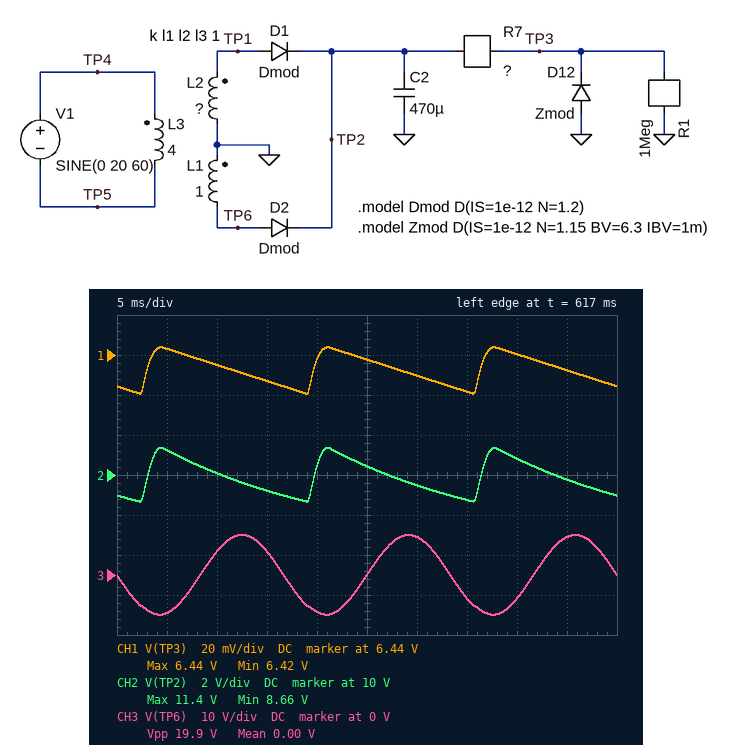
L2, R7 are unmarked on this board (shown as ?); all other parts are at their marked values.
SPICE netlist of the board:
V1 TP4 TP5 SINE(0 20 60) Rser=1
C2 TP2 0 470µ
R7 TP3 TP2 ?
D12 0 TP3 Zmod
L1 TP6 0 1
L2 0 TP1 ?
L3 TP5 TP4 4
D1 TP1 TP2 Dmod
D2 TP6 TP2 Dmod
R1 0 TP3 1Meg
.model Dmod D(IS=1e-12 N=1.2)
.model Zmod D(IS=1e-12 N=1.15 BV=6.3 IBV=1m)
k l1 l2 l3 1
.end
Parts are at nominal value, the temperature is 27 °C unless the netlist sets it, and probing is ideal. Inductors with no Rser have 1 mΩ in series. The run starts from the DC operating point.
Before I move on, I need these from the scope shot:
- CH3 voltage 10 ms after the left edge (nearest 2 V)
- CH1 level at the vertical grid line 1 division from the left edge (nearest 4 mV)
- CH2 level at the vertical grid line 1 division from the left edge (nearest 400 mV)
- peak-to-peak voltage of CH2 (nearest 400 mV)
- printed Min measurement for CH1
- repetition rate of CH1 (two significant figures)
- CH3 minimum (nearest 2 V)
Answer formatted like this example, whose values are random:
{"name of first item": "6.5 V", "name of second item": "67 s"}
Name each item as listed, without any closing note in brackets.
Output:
{"CH3 voltage 10 ms after the left edge": "6 V", "CH1 level at the vertical grid line 1 division from the left edge": "6.444 V", "CH2 level at the vertical grid line 1 division from the left edge": "11.2 V", "peak-to-peak voltage of CH2": "2.8 V", "printed Min measurement for CH1": "6.42 V", "repetition rate of CH1": "60 Hz", "CH3 minimum": "-10 V"}
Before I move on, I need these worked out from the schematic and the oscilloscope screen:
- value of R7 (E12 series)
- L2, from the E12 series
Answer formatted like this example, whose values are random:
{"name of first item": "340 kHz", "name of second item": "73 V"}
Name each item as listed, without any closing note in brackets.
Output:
{"value of R7": "39 Ω", "L2, from the E12 series": "1.5 H"}
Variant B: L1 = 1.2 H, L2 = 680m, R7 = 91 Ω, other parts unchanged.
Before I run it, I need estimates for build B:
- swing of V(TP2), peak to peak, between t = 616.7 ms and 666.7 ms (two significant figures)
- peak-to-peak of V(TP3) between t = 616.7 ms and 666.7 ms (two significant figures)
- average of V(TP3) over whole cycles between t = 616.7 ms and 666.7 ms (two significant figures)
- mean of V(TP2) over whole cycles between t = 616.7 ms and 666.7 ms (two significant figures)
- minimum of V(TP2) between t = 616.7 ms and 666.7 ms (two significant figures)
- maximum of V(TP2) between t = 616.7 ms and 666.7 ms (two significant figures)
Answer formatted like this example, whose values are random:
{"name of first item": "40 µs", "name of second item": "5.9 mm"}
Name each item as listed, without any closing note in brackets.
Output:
{"swing of V(TP2), peak to peak, between t = 616.7 ms and 666.7 ms": "1.1 V", "peak-to-peak of V(TP3) between t = 616.7 ms and 666.7 ms": "10 mV", "average of V(TP3) over whole cycles between t = 616.7 ms and 666.7 ms": "6.4 V", "mean of V(TP2) over whole cycles between t = 616.7 ms and 666.7 ms": "9.6 V", "minimum of V(TP2) between t = 616.7 ms and 666.7 ms": "9.0 V", "maximum of V(TP2) between t = 616.7 ms and 666.7 ms": "10 V"}
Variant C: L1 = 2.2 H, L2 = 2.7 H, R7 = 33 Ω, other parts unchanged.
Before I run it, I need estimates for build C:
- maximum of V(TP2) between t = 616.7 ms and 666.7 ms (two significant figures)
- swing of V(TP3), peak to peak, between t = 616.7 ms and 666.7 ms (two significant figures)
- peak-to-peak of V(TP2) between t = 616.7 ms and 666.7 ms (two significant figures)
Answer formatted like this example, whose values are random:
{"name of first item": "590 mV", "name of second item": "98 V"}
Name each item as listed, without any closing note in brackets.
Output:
{"maximum of V(TP2) between t = 616.7 ms and 666.7 ms": "15 V", "swing of V(TP3), peak to peak, between t = 616.7 ms and 666.7 ms": "17 mV", "peak-to-peak of V(TP2) between t = 616.7 ms and 666.7 ms": "3.8 V"}
